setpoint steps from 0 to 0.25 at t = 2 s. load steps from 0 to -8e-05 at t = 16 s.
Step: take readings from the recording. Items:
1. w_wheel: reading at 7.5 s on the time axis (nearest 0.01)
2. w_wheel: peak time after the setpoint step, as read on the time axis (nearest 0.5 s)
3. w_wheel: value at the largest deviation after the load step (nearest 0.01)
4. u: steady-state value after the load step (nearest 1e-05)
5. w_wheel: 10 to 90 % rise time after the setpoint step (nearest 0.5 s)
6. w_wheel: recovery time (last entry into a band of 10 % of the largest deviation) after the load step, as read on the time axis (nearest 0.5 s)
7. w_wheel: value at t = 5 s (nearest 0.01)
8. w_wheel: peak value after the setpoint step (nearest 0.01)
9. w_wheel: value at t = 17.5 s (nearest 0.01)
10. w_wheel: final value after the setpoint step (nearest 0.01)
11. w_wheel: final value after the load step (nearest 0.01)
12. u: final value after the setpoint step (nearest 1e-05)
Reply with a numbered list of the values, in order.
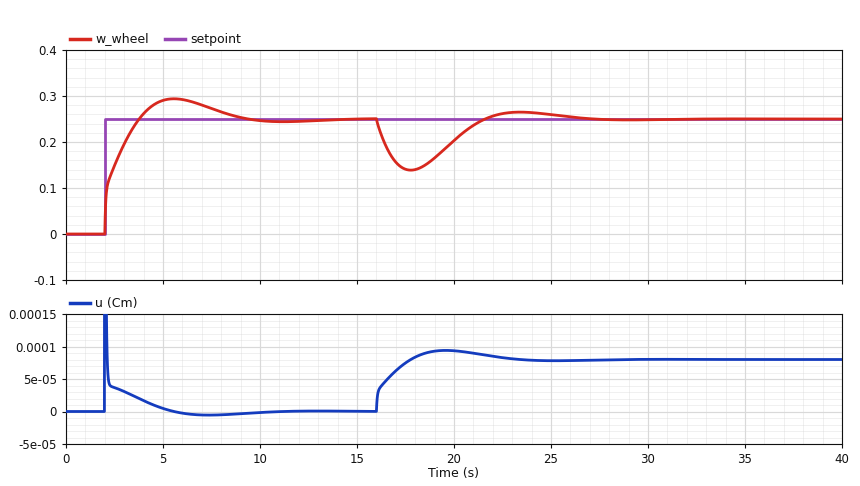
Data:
1. 0.27
2. 5.5 s
3. 0.14
4. 0.00008
5. 1.5 s
6. 24.5 s
7. 0.29
8. 0.29
9. 0.14
10. 0.25
11. 0.25
12. 0.00000
